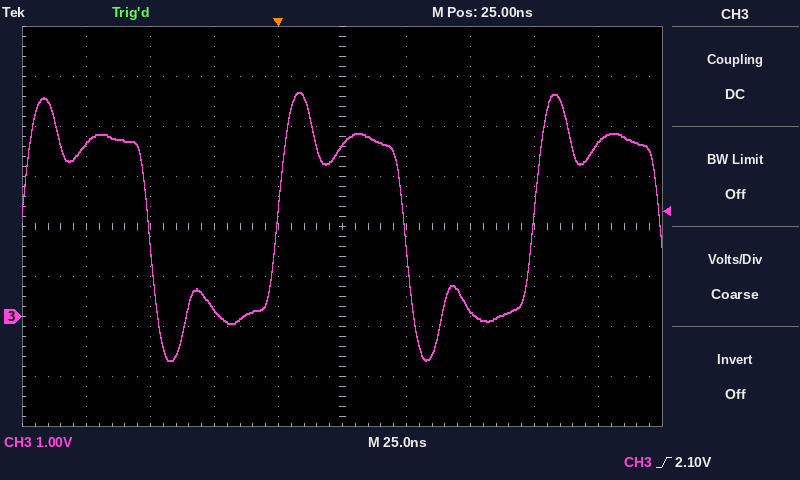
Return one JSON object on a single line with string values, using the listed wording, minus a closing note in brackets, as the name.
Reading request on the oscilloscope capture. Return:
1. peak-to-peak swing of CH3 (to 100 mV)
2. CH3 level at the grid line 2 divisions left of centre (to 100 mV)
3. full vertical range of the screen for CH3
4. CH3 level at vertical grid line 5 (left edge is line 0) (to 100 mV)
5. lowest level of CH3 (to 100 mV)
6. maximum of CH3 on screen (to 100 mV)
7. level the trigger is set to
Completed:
{"peak-to-peak swing of CH3": "5.4 V", "CH3 level at the grid line 2 divisions left of centre": "100 mV", "full vertical range of the screen for CH3": "8 V", "CH3 level at vertical grid line 5 (left edge is line 0)": "3.4 V", "lowest level of CH3": "-900 mV", "maximum of CH3 on screen": "4.5 V", "level the trigger is set to": "2.10 V"}
